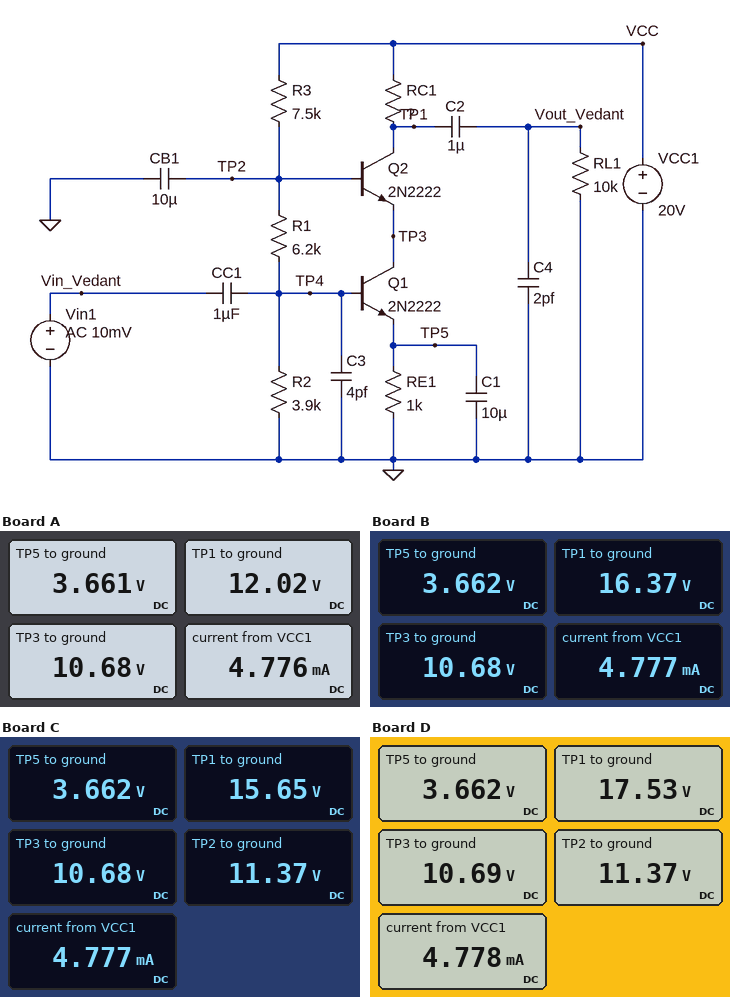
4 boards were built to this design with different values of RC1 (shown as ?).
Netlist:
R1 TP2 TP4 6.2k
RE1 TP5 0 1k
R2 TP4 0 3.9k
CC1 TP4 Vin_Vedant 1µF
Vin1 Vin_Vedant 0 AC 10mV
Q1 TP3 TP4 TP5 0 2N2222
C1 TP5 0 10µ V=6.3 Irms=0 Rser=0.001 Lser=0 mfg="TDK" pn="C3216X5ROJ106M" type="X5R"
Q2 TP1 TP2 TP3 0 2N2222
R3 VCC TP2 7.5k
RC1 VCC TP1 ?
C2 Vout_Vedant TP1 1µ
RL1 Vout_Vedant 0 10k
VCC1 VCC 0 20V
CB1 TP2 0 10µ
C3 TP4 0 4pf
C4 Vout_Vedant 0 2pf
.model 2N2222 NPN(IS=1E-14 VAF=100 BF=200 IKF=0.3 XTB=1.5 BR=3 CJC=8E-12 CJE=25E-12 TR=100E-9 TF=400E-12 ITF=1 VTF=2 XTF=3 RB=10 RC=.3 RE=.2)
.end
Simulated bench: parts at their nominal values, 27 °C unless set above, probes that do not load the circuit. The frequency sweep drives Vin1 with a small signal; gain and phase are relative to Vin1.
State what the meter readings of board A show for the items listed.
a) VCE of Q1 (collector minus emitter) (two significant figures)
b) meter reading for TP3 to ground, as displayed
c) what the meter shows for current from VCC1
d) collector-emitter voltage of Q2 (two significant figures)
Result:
7.0 V
10.68 V
4.776 mA
1.3 V
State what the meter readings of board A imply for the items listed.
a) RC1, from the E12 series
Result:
2.2 kΩ
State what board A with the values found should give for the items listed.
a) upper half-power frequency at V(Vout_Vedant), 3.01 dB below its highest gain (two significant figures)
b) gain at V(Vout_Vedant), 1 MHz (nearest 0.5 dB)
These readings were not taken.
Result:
10 MHz
47.5 dB
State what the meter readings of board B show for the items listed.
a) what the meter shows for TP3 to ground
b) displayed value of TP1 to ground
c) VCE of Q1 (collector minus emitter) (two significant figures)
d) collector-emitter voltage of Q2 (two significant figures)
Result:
10.68 V
16.37 V
7.0 V
5.7 V
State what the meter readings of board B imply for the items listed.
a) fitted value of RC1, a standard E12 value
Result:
1 kΩ
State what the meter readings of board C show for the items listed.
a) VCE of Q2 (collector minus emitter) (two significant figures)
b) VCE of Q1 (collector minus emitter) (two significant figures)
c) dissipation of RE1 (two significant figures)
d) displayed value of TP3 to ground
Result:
5.0 V
7.0 V
13 mW
10.68 V
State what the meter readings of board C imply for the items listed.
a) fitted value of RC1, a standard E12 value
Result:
1.2 kΩ
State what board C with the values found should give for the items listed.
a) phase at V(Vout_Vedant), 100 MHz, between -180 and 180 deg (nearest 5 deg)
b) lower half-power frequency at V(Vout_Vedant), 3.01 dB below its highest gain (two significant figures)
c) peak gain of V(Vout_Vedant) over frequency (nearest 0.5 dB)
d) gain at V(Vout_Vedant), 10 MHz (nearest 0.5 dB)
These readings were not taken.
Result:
45 deg
2.3 kHz
43.0 dB
42.5 dB
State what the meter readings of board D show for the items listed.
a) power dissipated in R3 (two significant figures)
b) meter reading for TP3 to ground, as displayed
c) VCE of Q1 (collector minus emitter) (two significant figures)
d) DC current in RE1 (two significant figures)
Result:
9.9 mW
10.69 V
7.0 V
3.7 mA
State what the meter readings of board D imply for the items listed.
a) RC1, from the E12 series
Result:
680 Ω
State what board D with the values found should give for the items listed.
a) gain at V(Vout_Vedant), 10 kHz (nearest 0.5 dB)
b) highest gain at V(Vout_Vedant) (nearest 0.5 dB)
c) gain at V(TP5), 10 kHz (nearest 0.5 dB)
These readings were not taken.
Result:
38.5 dB
38.5 dB
-13.5 dB
